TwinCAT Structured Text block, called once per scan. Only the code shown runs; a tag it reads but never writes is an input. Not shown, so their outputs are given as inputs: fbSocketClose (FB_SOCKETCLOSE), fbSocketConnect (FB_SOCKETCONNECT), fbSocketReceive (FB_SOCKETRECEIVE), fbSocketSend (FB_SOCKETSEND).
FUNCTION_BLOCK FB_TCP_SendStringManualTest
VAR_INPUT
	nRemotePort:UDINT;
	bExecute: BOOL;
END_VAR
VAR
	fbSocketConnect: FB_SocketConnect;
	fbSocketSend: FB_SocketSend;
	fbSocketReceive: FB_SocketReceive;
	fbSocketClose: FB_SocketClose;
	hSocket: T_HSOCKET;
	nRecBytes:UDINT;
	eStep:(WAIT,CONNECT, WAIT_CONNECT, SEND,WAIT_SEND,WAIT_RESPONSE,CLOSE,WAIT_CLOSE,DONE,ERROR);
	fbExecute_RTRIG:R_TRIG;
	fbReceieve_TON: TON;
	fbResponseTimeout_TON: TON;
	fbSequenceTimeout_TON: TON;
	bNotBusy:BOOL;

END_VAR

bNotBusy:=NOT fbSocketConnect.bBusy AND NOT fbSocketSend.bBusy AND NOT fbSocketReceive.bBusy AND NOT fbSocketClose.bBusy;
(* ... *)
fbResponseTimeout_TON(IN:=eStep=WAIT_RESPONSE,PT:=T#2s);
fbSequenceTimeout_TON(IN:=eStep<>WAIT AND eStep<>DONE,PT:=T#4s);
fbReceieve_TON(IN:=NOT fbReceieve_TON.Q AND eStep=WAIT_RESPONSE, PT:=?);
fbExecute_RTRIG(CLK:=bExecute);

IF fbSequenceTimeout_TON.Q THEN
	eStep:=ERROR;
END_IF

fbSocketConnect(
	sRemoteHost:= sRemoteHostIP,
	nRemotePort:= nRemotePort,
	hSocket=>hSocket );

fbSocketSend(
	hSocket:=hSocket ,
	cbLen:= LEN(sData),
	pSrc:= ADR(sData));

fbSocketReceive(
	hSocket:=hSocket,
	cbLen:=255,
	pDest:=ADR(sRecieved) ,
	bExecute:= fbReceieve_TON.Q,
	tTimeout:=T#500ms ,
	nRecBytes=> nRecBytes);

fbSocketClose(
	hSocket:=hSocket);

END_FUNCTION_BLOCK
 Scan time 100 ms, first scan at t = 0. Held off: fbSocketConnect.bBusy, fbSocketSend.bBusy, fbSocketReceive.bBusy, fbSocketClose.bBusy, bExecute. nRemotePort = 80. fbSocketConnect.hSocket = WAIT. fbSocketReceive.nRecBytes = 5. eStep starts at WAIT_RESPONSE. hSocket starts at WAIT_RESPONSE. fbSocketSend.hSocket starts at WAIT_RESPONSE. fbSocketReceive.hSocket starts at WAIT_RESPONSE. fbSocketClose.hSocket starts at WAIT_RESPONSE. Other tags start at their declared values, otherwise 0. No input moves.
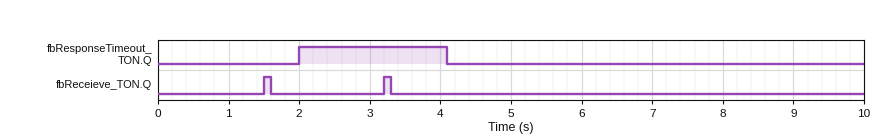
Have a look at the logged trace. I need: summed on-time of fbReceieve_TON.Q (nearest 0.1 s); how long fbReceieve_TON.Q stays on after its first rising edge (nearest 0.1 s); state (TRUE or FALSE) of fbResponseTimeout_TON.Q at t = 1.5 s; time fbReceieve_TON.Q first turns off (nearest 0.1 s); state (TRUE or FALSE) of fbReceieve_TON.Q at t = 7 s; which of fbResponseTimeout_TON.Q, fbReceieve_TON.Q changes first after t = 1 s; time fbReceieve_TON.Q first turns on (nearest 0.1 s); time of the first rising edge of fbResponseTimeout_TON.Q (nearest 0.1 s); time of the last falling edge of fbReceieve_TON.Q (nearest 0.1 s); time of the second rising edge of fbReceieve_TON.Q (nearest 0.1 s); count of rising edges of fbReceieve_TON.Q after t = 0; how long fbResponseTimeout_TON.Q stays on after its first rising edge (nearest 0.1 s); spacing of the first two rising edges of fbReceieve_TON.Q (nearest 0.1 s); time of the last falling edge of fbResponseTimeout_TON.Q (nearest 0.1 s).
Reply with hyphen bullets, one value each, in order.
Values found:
- 0.2 s
- 0.1 s
- FALSE
- 1.6 s
- FALSE
- fbReceieve_TON.Q
- 1.5 s
- 2.0 s
- 3.3 s
- 3.2 s
- 2
- 2.1 s
- 1.7 s
- 4.1 s
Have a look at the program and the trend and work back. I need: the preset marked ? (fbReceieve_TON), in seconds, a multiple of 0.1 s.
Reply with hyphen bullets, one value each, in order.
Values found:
- 1.5 s
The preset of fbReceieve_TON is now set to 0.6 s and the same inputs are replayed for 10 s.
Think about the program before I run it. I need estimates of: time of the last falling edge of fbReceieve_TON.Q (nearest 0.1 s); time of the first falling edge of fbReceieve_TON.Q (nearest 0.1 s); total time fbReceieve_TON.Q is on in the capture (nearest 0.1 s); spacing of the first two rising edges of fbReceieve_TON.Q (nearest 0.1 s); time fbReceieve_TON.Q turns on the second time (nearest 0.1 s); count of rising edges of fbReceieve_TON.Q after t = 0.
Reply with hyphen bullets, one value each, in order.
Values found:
- 3.9 s
- 0.7 s
- 0.5 s
- 0.8 s
- 1.4 s
- 5
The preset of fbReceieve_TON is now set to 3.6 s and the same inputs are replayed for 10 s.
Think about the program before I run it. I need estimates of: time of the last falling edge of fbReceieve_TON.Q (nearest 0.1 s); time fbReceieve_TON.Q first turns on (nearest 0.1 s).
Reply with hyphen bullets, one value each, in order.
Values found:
- 3.7 s
- 3.6 s
